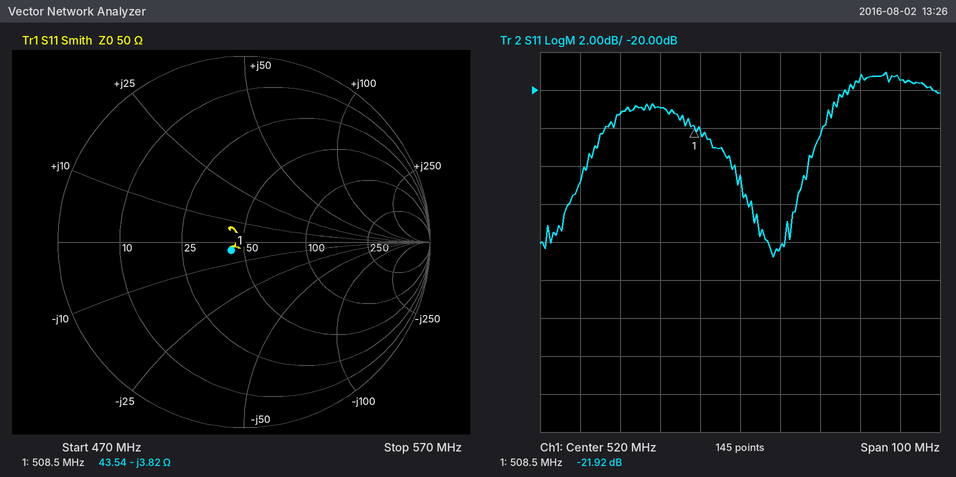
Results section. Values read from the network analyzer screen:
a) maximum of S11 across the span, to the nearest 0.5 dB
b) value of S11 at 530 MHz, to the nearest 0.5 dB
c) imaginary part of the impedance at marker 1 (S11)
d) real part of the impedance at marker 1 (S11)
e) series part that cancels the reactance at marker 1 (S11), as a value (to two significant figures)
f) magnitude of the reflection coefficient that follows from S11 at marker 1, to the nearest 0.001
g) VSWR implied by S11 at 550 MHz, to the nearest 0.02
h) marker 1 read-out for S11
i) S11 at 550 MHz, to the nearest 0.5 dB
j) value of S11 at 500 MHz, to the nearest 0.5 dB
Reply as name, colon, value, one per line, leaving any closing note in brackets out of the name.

maximum of S11 across the span, to the nearest 0.5 dB: -19.0 dB
value of S11 at 530 MHz, to the nearest 0.5 dB: -28.5 dB
imaginary part of the impedance at marker 1: -3.82 Ω
real part of the impedance at marker 1: 43.54 Ω
series part that cancels the reactance at marker 1 (S11), as a value: 1.2 nH
magnitude of the reflection coefficient that follows from S11 at marker 1, to the nearest 0.001: 0.080
VSWR implied by S11 at 550 MHz, to the nearest 0.02: 1.24
marker 1 read-out for S11: -21.92 dB
S11 at 550 MHz, to the nearest 0.5 dB: -19.5 dB
value of S11 at 500 MHz, to the nearest 0.5 dB: -21.0 dB
